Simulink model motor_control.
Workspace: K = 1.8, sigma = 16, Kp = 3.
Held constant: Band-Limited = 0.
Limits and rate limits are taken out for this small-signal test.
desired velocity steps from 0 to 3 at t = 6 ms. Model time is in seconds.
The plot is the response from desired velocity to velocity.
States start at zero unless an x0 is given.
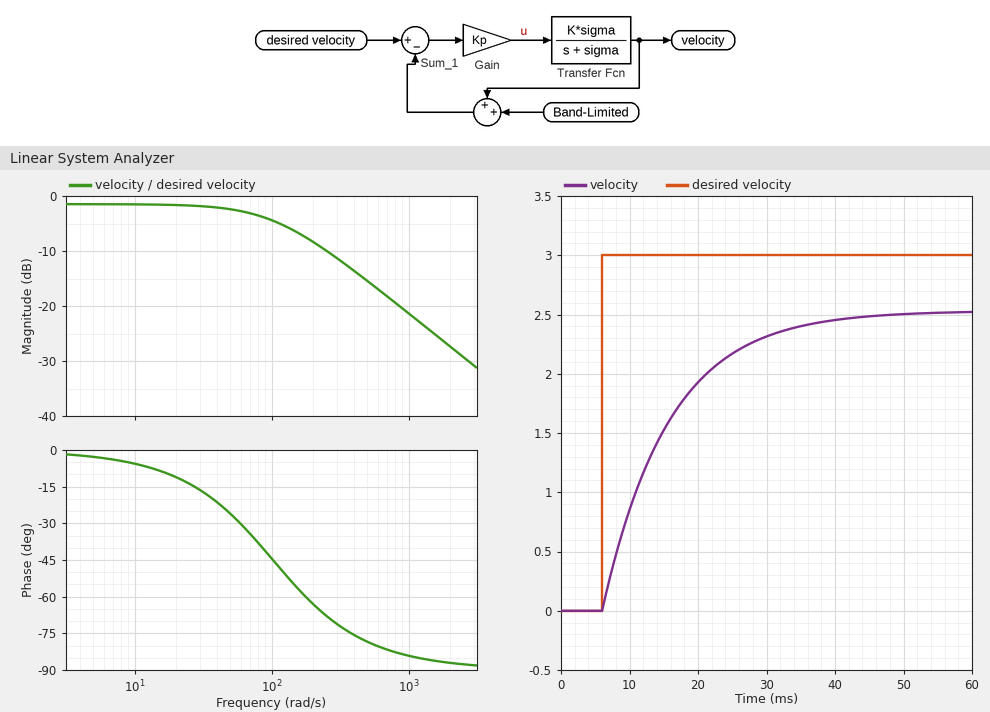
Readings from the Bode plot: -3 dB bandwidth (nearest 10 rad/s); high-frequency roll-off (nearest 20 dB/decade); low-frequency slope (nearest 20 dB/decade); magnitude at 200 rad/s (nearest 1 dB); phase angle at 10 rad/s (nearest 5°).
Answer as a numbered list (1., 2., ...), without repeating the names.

1. 100 rad/s
2. -20 dB/decade
3. 0 dB/decade
4. -8 dB
5. -5°
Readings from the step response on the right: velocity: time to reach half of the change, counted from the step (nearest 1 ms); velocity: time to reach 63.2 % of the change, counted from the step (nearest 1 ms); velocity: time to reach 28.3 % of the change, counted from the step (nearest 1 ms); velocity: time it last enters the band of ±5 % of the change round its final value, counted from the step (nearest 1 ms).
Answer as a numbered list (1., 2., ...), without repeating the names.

1. 7 ms
2. 10 ms
3. 3 ms
4. 29 ms
